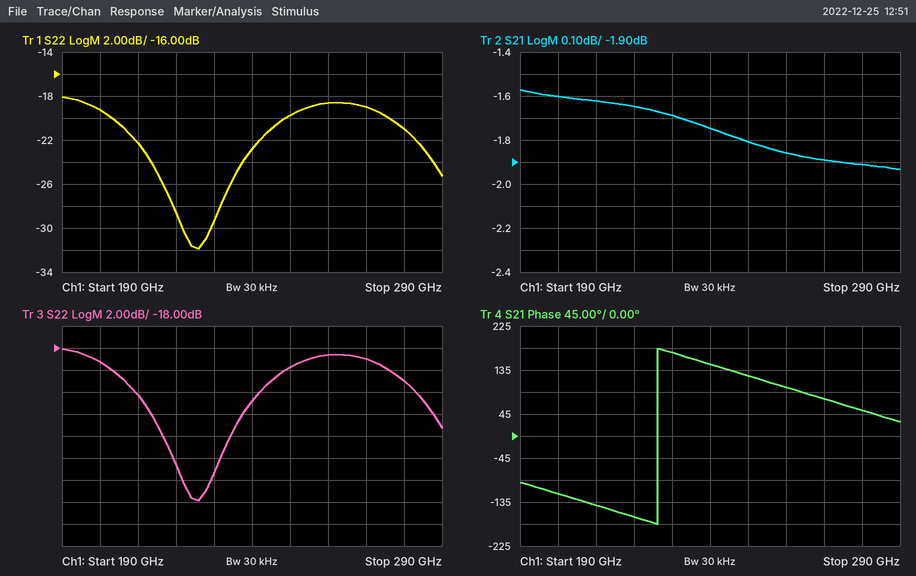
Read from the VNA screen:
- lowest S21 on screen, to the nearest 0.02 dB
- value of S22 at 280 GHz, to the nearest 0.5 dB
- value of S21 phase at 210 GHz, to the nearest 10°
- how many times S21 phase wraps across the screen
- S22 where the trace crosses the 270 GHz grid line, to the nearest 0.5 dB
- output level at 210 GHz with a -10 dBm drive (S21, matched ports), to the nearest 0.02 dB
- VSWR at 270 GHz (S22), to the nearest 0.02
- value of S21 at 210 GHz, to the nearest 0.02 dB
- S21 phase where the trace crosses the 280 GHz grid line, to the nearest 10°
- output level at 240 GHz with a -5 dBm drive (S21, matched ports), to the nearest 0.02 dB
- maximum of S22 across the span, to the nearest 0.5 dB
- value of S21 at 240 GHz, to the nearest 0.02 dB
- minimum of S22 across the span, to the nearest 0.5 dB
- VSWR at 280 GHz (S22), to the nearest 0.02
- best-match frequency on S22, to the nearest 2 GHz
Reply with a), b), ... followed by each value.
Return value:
a) -1.94 dB
b) -21.0 dB
c) -140°
d) 1
e) -19.0 dB
f) -11.62 dBm
g) 1.26
h) -1.62 dB
i) 50°
j) -6.74 dBm
k) -18.0 dB
l) -1.74 dB
m) -32.0 dB
n) 1.20
o) 226 GHz
